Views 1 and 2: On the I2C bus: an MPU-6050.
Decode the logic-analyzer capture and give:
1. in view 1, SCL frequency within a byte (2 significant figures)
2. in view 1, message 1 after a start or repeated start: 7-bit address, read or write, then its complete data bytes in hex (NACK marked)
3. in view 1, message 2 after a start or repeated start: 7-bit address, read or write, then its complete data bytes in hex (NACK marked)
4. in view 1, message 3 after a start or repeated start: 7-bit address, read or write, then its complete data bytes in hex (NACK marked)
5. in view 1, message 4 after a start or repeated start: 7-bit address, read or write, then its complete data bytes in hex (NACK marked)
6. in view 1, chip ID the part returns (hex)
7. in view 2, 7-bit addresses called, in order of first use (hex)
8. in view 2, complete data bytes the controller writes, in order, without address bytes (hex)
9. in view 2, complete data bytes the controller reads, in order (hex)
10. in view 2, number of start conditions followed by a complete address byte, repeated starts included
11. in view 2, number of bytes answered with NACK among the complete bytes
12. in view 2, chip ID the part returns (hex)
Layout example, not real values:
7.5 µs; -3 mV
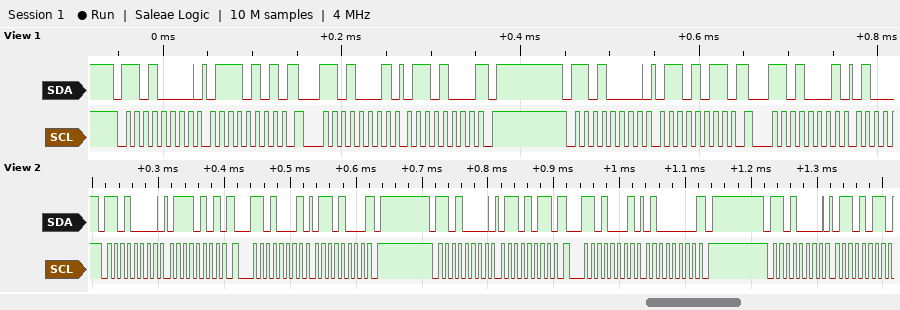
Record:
100 kHz; 0x68 write: 75; 0x68 read: 68 NACK; 0x68 write: 6B; 0x68 read; 0x68; 0x68; 75 6B 6B; 68 40; 5; 2; 0x68
